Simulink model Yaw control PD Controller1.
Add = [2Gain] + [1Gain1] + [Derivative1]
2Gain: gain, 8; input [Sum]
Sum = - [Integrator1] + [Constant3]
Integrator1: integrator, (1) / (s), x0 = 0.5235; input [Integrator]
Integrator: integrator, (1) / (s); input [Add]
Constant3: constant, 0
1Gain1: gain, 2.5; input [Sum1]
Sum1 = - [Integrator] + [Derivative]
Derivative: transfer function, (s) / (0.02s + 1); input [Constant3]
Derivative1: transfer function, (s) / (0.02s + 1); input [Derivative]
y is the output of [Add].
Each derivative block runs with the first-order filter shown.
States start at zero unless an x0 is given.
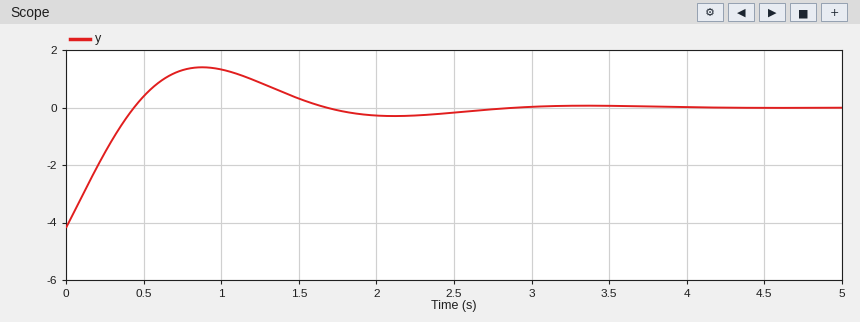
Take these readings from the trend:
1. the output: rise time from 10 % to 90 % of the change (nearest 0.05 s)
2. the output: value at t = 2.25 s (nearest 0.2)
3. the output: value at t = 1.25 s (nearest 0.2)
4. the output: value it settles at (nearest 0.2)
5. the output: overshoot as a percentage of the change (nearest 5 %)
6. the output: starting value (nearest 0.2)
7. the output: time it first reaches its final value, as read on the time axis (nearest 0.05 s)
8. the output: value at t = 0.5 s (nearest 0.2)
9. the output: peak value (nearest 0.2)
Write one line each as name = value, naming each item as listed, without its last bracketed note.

the output: rise time from 10 % to 90 % of the change = 0.35 s
the output: value at t = 2.25 s = -0.2
the output: value at t = 1.25 s = 0.8
the output: value it settles at = 0.0
the output: overshoot as a percentage of the change = 35 %
the output: starting value = -4.2
the output: time it first reaches its final value, as read on the time axis = 0.45 s
the output: value at t = 0.5 s = 0.4
the output: peak value = 1.4
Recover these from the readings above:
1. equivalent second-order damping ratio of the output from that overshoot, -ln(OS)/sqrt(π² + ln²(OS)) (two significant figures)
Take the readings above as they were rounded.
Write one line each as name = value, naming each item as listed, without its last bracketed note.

equivalent second-order damping ratio of the output from that overshoot, -ln(OS)/sqrt(π² + ln²(OS)) = 0.32
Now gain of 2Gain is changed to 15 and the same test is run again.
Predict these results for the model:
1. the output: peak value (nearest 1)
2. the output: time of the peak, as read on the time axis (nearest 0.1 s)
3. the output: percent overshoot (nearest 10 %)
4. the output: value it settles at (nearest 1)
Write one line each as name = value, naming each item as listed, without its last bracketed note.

the output: peak value = 3
the output: time of the peak, as read on the time axis = 0.7 s
the output: percent overshoot = 40 %
the output: value it settles at = 0
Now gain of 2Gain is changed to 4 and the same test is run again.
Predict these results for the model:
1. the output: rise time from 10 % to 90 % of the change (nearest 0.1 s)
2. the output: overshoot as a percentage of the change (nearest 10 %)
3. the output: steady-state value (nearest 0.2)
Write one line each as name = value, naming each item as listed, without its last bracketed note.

the output: rise time from 10 % to 90 % of the change = 0.4 s
the output: overshoot as a percentage of the change = 20 %
the output: steady-state value = 0.0
